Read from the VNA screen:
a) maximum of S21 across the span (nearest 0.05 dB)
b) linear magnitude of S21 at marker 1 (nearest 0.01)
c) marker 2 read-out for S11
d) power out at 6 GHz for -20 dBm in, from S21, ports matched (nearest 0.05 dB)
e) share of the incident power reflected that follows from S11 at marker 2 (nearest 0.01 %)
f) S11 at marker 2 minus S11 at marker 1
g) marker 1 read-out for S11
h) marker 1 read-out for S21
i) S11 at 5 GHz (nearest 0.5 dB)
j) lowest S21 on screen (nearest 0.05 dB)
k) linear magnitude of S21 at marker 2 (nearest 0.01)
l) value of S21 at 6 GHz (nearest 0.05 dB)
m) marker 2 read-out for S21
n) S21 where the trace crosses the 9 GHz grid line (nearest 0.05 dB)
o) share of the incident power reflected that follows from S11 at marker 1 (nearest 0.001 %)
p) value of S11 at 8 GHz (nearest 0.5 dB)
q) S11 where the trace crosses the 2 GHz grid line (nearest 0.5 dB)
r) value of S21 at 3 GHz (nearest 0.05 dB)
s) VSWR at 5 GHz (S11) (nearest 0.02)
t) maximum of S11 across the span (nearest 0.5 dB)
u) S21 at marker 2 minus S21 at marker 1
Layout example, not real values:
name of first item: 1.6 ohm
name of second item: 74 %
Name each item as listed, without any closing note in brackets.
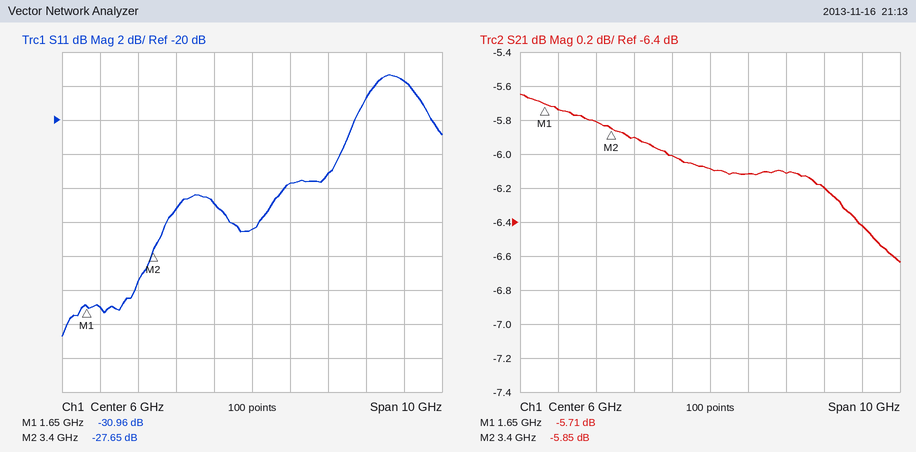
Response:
maximum of S21 across the span: -5.65 dB
linear magnitude of S21 at marker 1: 0.52
marker 2 read-out for S11: -27.65 dB
power out at 6 GHz for -20 dBm in, from S21, ports matched: -26.10 dBm
share of the incident power reflected that follows from S11 at marker 2: 0.17 %
S11 at marker 2 minus S11 at marker 1: 3.31 dB
marker 1 read-out for S11: -30.96 dB
marker 1 read-out for S21: -5.71 dB
S11 at 5 GHz: -25.0 dB
lowest S21 on screen: -6.65 dB
linear magnitude of S21 at marker 2: 0.51
value of S21 at 6 GHz: -6.10 dB
marker 2 read-out for S21: -5.85 dB
S21 where the trace crosses the 9 GHz grid line: -6.20 dB
share of the incident power reflected that follows from S11 at marker 1: 0.080 %
value of S11 at 8 GHz: -23.0 dB
S11 where the trace crosses the 2 GHz grid line: -31.0 dB
value of S21 at 3 GHz: -5.80 dB
VSWR at 5 GHz (S11): 1.12
maximum of S11 across the span: -17.5 dB
S21 at marker 2 minus S21 at marker 1: -0.14 dB
